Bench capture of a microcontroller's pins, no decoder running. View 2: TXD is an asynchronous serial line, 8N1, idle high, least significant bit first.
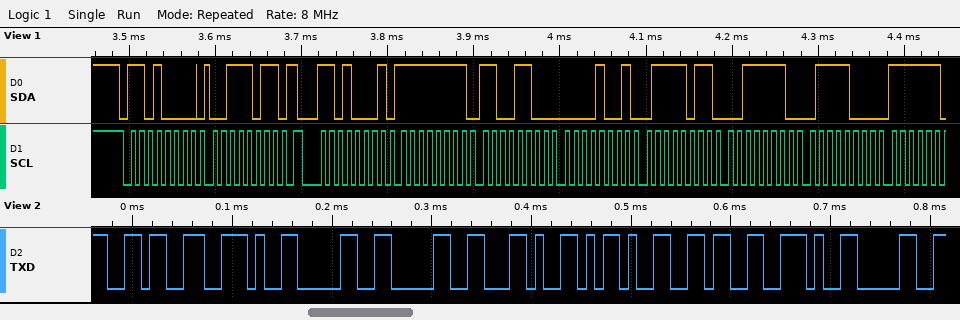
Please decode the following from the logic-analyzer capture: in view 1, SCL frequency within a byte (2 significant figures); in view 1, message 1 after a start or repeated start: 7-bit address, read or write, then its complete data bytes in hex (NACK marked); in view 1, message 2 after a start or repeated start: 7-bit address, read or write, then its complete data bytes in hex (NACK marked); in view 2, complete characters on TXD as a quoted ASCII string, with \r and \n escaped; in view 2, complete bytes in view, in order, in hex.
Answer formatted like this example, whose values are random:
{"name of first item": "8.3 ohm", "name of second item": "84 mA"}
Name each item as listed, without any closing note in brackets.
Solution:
{"in view 1, SCL frequency within a byte": "100 kHz", "in view 1, message 1 after a start or repeated start: 7-bit address, read or write, then its complete data bytes in hex": "0x68 write: 3B", "in view 1, message 2 after a start or repeated start: 7-bit address, read or write, then its complete data bytes in hex": "0x68 read: FF CC 09 7B 3E 78", "in view 2, complete characters on TXD as a quoted ASCII string, with \\r and \\n escaped": "\"6.00,-6.0\"", "in view 2, complete bytes in view, in order, in hex": "0x36 0x2E 0x30 0x30 0x2C 0x2D 0x36 0x2E 0x30"}
